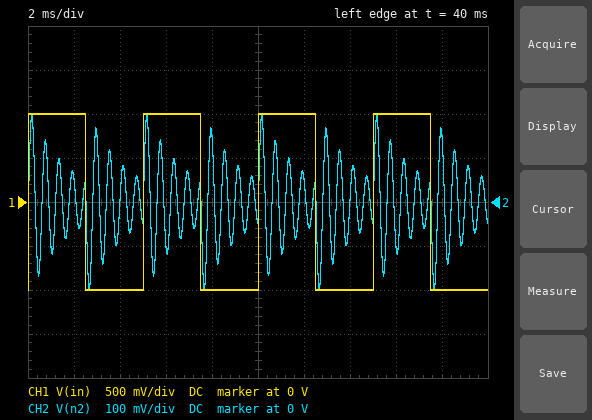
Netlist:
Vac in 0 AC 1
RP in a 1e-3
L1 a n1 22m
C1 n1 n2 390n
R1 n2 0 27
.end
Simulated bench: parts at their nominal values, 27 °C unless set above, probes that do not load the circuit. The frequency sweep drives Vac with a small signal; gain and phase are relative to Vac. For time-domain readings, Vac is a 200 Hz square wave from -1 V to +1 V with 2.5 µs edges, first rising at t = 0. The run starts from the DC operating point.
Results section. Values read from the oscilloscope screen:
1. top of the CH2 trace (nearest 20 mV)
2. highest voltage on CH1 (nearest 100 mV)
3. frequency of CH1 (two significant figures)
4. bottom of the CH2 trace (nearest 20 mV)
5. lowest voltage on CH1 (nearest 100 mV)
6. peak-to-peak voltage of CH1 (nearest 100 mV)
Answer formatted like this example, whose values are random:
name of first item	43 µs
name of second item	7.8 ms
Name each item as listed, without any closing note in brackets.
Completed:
top of the CH2 trace	200 mV
highest voltage on CH1	1.0 V
frequency of CH1	200 Hz
bottom of the CH2 trace	-200 mV
lowest voltage on CH1	-1.0 V
peak-to-peak voltage of CH1	2.0 V
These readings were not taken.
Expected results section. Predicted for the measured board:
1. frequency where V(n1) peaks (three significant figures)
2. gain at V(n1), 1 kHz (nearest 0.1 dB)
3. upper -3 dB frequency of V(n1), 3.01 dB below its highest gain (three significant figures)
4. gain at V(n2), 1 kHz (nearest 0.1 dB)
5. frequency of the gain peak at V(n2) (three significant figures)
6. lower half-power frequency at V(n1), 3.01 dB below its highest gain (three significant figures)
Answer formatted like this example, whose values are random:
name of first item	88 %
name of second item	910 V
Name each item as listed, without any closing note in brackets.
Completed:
frequency where V(n1) peaks	1.71 kHz
gain at V(n1), 1 kHz	3.6 dB
upper -3 dB frequency of V(n1), 3.01 dB below its highest gain	1.81 kHz
gain at V(n2), 1 kHz	-20.0 dB
frequency of the gain peak at V(n2)	1.72 kHz
lower half-power frequency at V(n1), 3.01 dB below its highest gain	1.61 kHz
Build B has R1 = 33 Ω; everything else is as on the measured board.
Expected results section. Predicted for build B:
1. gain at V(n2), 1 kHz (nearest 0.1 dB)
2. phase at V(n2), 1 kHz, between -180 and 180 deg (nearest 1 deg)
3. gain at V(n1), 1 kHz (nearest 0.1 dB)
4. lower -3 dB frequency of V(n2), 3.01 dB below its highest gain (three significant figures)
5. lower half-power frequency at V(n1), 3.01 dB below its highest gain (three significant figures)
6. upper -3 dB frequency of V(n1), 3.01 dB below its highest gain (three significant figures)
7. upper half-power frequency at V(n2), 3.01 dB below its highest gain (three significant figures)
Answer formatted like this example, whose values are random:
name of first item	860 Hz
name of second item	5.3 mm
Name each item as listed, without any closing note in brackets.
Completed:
gain at V(n2), 1 kHz	-18.3 dB
phase at V(n2), 1 kHz, between -180 and 180 deg	83 deg
gain at V(n1), 1 kHz	3.6 dB
lower -3 dB frequency of V(n2), 3.01 dB below its highest gain	1.60 kHz
lower half-power frequency at V(n1), 3.01 dB below its highest gain	1.59 kHz
upper -3 dB frequency of V(n1), 3.01 dB below its highest gain	1.83 kHz
upper half-power frequency at V(n2), 3.01 dB below its highest gain	1.84 kHz
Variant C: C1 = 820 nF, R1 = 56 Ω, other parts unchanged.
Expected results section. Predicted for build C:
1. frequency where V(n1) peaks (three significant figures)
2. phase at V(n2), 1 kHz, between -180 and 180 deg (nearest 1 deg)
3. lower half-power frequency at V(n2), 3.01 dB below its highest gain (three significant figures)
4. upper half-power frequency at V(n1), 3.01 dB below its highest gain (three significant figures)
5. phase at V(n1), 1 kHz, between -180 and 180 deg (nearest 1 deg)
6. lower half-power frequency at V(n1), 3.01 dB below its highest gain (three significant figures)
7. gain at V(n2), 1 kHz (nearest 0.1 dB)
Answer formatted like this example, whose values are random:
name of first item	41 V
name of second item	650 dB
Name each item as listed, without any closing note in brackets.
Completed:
frequency where V(n1) peaks	1.15 kHz
phase at V(n2), 1 kHz, between -180 and 180 deg	45 deg
lower half-power frequency at V(n2), 3.01 dB below its highest gain	1.00 kHz
upper half-power frequency at V(n1), 3.01 dB below its highest gain	1.35 kHz
phase at V(n1), 1 kHz, between -180 and 180 deg	-29 deg
lower half-power frequency at V(n1), 3.01 dB below its highest gain	930 Hz
gain at V(n2), 1 kHz	-3.0 dB
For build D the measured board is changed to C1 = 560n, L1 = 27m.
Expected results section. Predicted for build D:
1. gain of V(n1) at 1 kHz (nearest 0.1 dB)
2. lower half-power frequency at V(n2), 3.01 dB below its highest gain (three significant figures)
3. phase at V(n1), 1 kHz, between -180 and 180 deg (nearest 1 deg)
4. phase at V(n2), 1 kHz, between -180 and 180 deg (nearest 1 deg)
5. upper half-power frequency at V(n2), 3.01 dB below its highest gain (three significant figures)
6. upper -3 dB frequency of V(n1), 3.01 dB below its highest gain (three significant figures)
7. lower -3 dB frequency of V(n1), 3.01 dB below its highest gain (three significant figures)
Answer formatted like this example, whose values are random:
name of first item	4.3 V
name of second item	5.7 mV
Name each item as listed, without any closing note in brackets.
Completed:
gain of V(n1) at 1 kHz	7.7 dB
lower half-power frequency at V(n2), 3.01 dB below its highest gain	1.22 kHz
phase at V(n1), 1 kHz, between -180 and 180 deg	-8 deg
phase at V(n2), 1 kHz, between -180 and 180 deg	77 deg
upper half-power frequency at V(n2), 3.01 dB below its highest gain	1.38 kHz
upper -3 dB frequency of V(n1), 3.01 dB below its highest gain	1.37 kHz
lower -3 dB frequency of V(n1), 3.01 dB below its highest gain	1.21 kHz
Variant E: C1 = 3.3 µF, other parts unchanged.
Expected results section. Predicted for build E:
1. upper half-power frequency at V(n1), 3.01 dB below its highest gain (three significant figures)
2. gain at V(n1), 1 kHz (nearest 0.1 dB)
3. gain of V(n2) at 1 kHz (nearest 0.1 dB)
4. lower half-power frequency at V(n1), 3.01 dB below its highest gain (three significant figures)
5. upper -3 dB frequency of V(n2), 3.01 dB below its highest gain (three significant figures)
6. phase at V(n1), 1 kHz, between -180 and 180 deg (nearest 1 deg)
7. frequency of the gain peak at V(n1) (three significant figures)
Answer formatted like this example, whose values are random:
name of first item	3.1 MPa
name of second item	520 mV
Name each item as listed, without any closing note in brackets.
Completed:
upper half-power frequency at V(n1), 3.01 dB below its highest gain	669 Hz
gain at V(n1), 1 kHz	-4.6 dB
gain of V(n2) at 1 kHz	-10.8 dB
lower half-power frequency at V(n1), 3.01 dB below its highest gain	469 Hz
upper -3 dB frequency of V(n2), 3.01 dB below its highest gain	696 Hz
phase at V(n1), 1 kHz, between -180 and 180 deg	-134 deg
frequency of the gain peak at V(n1)	576 Hz
